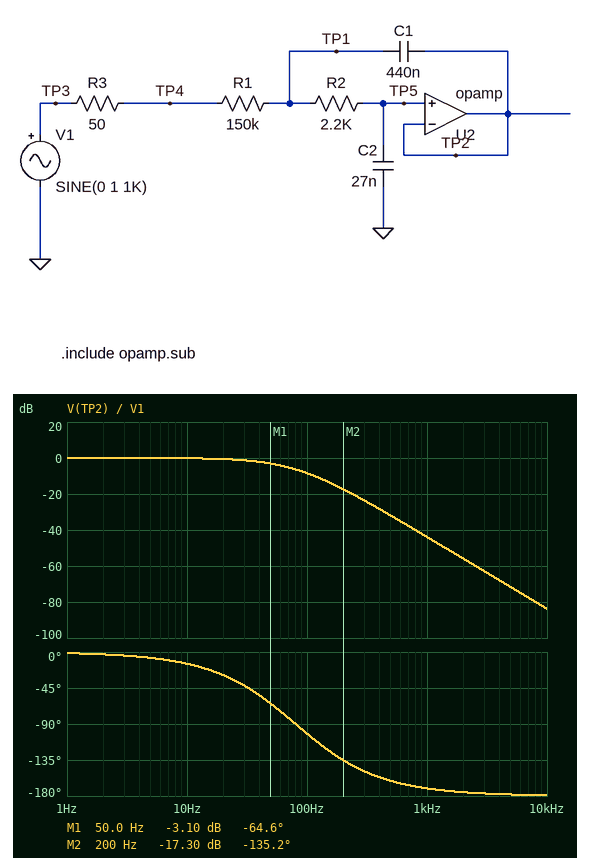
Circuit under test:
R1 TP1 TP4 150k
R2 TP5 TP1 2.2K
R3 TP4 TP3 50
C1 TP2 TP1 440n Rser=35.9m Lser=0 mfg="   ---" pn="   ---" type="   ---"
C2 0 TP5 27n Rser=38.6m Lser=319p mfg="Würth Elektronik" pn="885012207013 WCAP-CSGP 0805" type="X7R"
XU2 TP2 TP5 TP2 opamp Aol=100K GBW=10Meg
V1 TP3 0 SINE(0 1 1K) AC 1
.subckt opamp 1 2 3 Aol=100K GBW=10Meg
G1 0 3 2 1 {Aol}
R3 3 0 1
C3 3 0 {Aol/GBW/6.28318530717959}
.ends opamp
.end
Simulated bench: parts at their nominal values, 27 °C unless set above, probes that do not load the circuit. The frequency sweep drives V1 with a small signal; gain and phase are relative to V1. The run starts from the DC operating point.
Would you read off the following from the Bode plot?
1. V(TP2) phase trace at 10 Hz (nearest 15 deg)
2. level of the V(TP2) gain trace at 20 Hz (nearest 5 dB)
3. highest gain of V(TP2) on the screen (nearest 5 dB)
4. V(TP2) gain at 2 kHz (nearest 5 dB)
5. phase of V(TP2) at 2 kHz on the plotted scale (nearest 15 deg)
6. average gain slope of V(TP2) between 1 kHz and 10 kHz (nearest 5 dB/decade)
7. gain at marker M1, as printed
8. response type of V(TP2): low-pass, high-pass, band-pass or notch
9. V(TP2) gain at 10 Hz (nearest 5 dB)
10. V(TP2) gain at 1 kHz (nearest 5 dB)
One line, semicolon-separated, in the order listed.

-15 deg; 0 dB; 0 dB; -55 dB; -180 deg; -40 dB/decade; -3.10 dB; low-pass; 0 dB; -45 dB
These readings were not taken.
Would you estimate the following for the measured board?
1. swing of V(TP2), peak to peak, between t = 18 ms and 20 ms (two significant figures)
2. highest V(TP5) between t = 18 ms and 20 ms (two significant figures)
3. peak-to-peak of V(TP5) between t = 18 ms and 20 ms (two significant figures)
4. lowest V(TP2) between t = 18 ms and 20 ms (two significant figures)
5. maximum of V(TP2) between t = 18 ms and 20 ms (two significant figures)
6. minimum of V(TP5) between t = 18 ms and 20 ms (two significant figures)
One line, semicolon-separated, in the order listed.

13 mV; 6.5 mV; 13 mV; -6.3 mV; 6.5 mV; -6.3 mV
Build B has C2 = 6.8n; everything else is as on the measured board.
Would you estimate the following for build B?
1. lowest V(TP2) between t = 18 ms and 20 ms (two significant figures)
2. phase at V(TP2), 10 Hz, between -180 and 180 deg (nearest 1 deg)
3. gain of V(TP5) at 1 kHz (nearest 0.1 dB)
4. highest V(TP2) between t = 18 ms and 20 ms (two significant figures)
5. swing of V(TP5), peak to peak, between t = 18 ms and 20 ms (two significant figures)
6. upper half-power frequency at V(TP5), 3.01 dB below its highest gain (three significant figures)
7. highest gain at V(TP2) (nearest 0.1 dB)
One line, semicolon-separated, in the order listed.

-26 mV; -4 deg; -31.7 dB; 26 mV; 52 mV; 186 Hz; 1.0 dB
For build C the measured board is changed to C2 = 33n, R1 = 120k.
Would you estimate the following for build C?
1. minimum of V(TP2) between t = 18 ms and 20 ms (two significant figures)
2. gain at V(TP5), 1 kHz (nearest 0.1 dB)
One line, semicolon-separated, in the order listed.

-6.5 mV; -43.7 dB
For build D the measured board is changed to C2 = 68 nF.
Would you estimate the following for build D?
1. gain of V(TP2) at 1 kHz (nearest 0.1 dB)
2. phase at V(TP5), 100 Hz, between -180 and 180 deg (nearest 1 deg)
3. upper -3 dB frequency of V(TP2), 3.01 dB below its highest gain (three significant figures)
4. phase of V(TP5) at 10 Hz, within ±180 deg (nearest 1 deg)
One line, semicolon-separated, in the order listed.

-51.9 dB; -114 deg; 16.9 Hz; -34 deg
